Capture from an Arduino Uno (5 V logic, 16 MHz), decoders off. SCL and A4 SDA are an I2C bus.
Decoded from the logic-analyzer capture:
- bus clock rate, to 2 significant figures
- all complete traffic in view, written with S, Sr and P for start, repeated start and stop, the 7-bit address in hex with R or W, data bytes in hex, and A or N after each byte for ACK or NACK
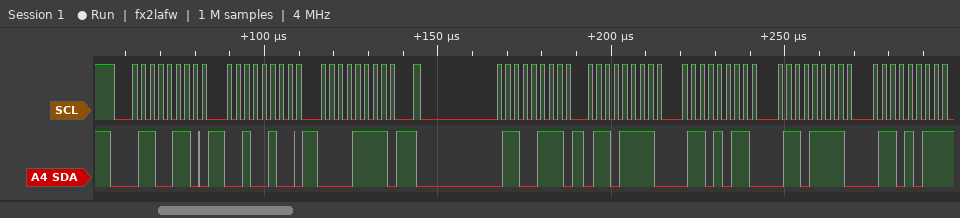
400 kHz
S 33W A 24 A 0F A Sr 33R A 6F A 6B A 6F A 6B N
